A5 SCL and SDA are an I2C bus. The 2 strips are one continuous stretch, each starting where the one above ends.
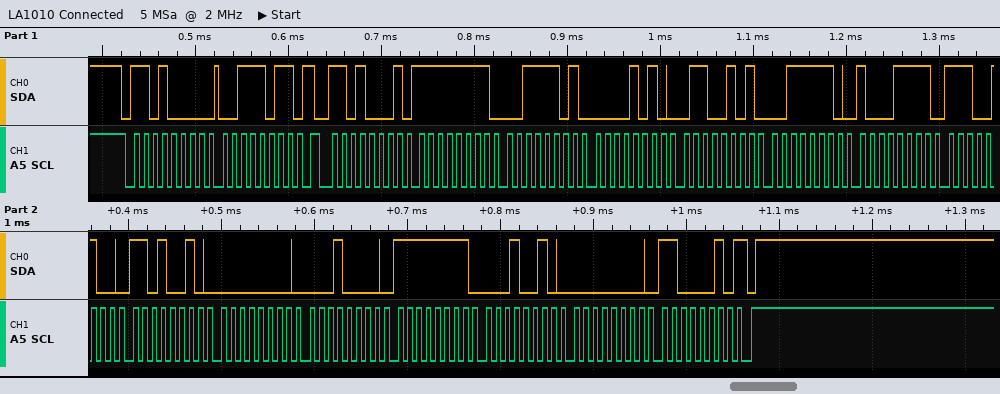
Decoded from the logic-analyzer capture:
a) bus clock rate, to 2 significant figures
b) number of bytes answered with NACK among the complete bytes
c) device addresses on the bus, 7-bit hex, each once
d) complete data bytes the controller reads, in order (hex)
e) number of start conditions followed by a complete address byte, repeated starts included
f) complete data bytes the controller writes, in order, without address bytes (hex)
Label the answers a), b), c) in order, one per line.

a) 100 kHz
b) 1
c) 0x68
d) FF 3D 0A 65 3E 8F E4 D2 00 10 FF 12 00 C2
e) 2
f) 3B
